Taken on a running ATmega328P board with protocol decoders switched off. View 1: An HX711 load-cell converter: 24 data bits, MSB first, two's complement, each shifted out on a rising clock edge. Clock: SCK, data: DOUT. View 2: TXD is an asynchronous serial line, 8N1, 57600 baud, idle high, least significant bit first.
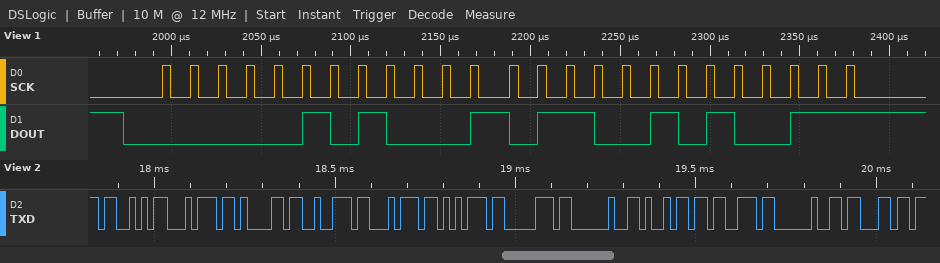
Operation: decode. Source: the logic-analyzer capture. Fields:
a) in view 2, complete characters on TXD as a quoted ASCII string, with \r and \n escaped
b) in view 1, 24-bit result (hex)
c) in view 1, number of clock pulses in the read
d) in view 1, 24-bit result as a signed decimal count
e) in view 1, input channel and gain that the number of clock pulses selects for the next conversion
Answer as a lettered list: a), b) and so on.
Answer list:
a) "Startup is c"
b) 0x051653
c) 25
d) 333395
e) channel A, gain 128
